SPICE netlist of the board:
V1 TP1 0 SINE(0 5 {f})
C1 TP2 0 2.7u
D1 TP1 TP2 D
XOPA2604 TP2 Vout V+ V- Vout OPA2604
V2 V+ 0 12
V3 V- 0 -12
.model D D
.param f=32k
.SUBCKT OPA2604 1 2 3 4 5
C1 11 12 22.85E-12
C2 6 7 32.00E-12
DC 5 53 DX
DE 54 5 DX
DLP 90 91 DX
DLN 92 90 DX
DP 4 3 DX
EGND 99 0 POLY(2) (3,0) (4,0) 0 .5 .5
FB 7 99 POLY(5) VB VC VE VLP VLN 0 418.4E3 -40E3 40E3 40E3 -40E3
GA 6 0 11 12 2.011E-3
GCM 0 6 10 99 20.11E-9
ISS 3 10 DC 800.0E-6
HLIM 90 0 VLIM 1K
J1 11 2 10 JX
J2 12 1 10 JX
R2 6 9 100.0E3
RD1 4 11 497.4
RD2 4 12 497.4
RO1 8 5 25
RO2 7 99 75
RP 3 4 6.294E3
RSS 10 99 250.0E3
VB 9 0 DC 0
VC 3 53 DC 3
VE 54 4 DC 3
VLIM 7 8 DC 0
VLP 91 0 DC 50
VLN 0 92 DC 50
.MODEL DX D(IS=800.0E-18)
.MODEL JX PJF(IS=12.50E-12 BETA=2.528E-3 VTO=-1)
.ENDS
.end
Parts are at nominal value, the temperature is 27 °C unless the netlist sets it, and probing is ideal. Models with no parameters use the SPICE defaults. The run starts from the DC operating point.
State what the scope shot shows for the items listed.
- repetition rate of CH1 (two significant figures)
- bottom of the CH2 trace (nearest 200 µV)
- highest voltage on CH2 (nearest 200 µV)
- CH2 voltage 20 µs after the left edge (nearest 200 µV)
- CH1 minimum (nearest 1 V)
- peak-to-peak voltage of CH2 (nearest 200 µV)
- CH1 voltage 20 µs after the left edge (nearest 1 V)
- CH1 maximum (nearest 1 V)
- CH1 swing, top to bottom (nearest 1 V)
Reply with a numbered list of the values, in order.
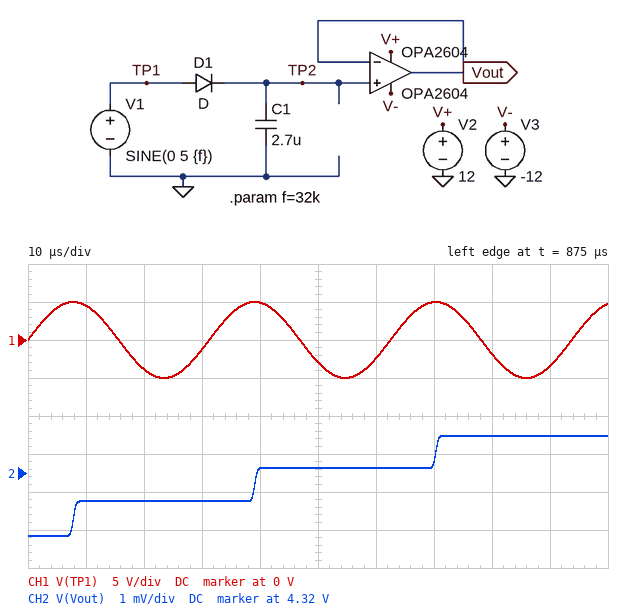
1. 32 kHz
2. 4.3184 V
3. 4.3210 V
4. 4.3192 V
5. -5 V
6. 2.6 mV
7. -4 V
8. 5 V
9. 10 V
